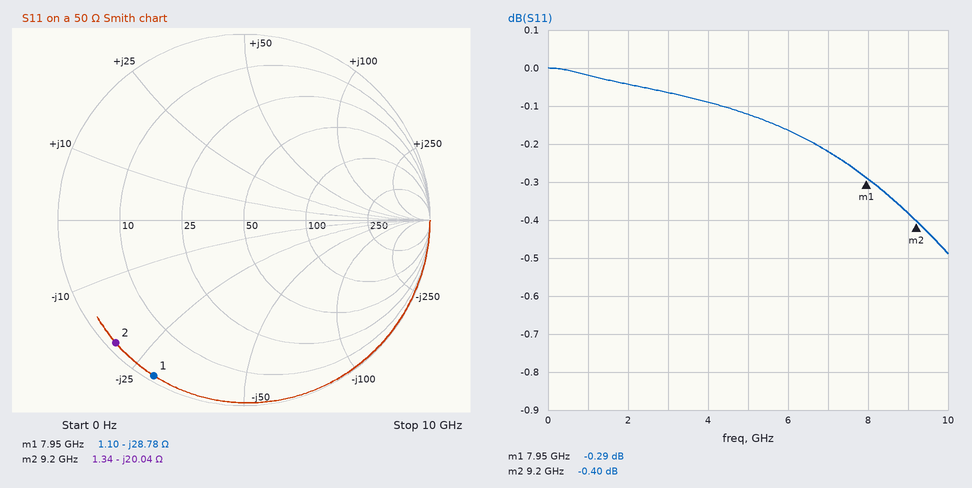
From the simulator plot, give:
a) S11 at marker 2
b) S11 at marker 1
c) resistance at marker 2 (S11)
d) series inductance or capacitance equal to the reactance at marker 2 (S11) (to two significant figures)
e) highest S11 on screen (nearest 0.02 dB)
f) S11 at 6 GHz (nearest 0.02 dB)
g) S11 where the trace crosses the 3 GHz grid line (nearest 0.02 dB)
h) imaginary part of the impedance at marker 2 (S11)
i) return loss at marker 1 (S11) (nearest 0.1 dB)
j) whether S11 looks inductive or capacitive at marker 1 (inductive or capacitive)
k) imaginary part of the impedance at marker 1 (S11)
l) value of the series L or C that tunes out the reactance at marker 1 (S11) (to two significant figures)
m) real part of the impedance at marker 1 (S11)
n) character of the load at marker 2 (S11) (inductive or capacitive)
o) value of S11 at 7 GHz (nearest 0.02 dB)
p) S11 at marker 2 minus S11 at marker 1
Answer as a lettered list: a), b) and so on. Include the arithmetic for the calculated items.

a) -0.40 dB
b) -0.29 dB
c) 1.34 Ω
d) C = 1/(2π × 9.2 GHz × 20.04 Ω) ≈ 863 fF, so 860 fF to two significant figures
e) 0.00 dB
f) -0.16 dB
g) -0.06 dB
h) -20.04 Ω
i) 0.3 dB
j) capacitive
k) -28.78 Ω
l) L = 28.78 Ω/(2π × 7.95 GHz) ≈ 576 pH, so 580 pH to two significant figures
m) 1.10 Ω
n) capacitive
o) -0.22 dB
p) -0.4 − (-0.29) = -0.11 dB
